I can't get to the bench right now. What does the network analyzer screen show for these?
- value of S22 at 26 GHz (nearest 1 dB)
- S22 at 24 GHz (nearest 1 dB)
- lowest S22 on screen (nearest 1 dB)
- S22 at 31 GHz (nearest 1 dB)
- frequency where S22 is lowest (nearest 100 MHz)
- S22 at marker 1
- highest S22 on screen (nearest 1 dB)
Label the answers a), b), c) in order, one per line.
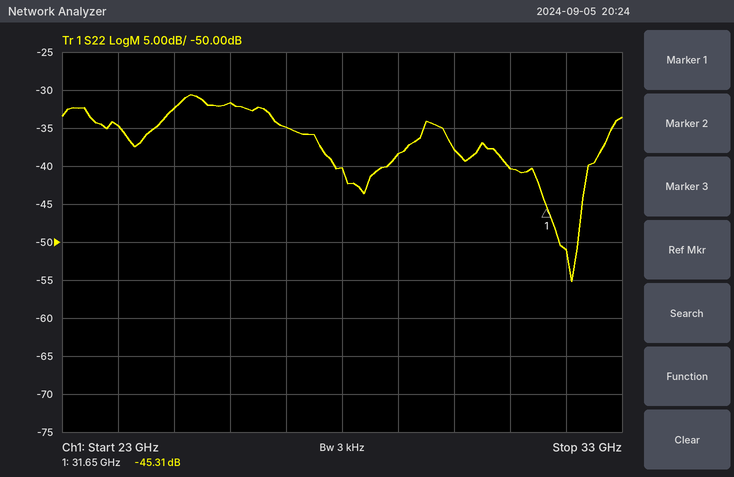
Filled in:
a) -32 dB
b) -35 dB
c) -55 dB
d) -40 dB
e) 32.1 GHz
f) -45.31 dB
g) -31 dB
